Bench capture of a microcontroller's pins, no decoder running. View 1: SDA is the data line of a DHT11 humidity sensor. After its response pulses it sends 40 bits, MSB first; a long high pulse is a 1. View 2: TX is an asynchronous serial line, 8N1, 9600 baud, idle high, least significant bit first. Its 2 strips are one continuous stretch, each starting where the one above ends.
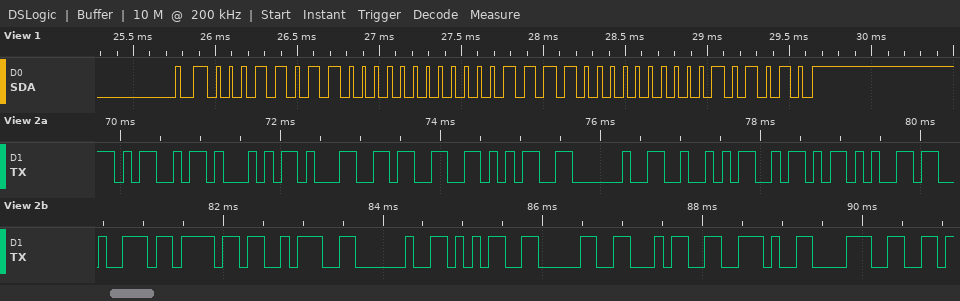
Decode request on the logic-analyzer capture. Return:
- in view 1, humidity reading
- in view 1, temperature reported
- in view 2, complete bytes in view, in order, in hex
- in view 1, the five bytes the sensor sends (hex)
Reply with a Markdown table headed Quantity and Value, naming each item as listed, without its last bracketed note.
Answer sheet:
| Quantity | Value |
|---|---|
| in view 1, humidity reading | 27 % |
| in view 1, temperature reported | 15.0 °C |
| in view 2, complete bytes in view, in order, in hex | 4D 51 31 33 35 20 52 5A 65 72 6F 3A 20 35 30 34 2E 38 |
| in view 1, the five bytes the sensor sends | 1B 00 0F 00 2A |
